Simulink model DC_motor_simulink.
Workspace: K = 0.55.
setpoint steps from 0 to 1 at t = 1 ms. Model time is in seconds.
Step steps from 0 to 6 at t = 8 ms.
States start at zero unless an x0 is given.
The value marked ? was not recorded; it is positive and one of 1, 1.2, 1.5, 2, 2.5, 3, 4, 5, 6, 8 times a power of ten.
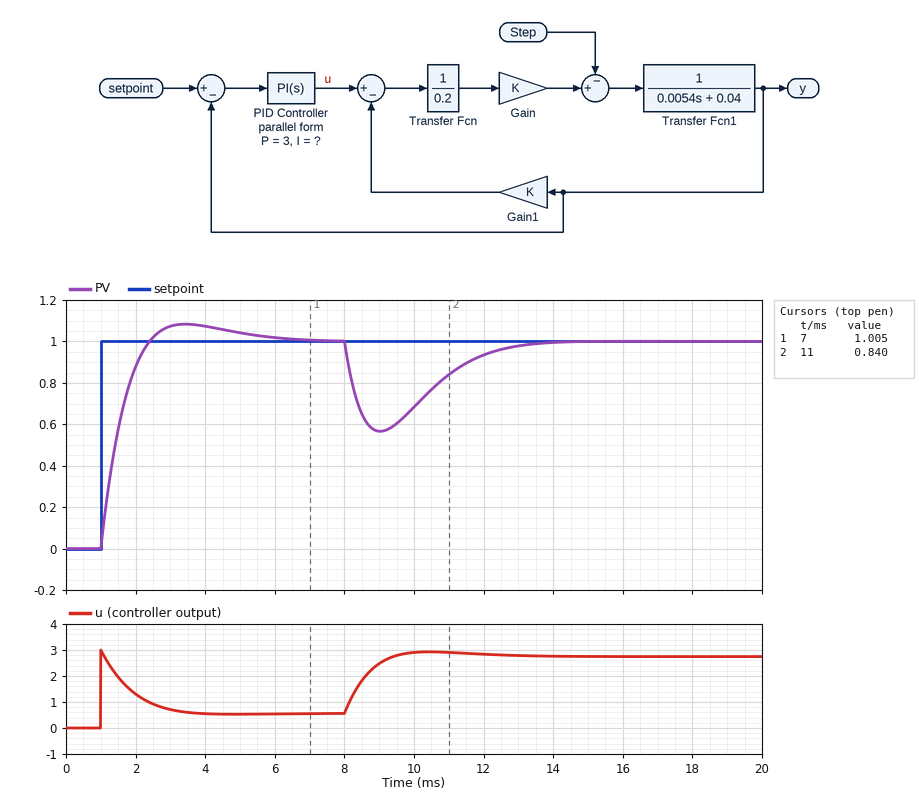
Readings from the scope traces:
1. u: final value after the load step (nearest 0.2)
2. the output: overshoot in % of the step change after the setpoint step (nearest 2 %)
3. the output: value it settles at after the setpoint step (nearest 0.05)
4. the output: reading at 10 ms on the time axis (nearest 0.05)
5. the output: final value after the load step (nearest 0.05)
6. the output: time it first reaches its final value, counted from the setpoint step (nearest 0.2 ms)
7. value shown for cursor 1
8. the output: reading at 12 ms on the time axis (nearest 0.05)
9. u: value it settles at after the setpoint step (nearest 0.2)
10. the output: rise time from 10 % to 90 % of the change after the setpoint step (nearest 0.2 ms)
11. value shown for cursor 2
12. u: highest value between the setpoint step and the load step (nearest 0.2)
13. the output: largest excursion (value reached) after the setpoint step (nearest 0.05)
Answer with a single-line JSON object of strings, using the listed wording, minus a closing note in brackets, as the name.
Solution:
{"u: final value after the load step": "2.8", "the output: overshoot in % of the step change after the setpoint step": "8 %", "the output: value it settles at after the setpoint step": "1.00", "the output: reading at 10 ms on the time axis": "0.70", "the output: final value after the load step": "1.00", "the output: time it first reaches its final value, counted from the setpoint step": "1.4 ms", "value shown for cursor 1": "1.005", "the output: reading at 12 ms on the time axis": "0.95", "u: value it settles at after the setpoint step": "0.6", "the output: rise time from 10 % to 90 % of the change after the setpoint step": "1.0 ms", "value shown for cursor 2": "0.840", "u: highest value between the setpoint step and the load step": "3.0", "the output: largest excursion (value reached) after the setpoint step": "1.10"}
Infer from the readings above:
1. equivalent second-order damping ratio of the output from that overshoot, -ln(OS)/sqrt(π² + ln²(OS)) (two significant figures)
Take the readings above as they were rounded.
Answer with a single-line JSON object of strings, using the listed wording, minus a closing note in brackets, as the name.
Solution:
{"equivalent second-order damping ratio of the output from that overshoot, -ln(OS)/sqrt(π² + ln²(OS))": "0.63"}
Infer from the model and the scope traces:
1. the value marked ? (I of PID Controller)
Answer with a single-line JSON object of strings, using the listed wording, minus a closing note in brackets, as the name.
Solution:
{"the value marked ?": "2000"}
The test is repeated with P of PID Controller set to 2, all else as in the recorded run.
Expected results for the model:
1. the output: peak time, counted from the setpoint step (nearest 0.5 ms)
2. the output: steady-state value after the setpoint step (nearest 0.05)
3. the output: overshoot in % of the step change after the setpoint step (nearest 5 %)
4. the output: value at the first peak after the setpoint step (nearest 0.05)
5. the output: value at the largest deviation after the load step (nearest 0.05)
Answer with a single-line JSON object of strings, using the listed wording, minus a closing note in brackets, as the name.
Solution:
{"the output: peak time, counted from the setpoint step": "2.5 ms", "the output: steady-state value after the setpoint step": "1.00", "the output: overshoot in % of the step change after the setpoint step": "15 %", "the output: value at the first peak after the setpoint step": "1.15", "the output: value at the largest deviation after the load step": "0.45"}
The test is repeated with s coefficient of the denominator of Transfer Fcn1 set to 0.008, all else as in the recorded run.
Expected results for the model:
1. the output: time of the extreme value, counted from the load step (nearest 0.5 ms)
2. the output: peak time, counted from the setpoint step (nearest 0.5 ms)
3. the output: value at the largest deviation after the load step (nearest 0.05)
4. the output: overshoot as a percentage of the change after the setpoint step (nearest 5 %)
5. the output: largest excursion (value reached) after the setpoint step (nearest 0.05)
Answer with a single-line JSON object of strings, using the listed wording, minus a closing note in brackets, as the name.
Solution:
{"the output: time of the extreme value, counted from the load step": "1.5 ms", "the output: peak time, counted from the setpoint step": "3.0 ms", "the output: value at the largest deviation after the load step": "0.60", "the output: overshoot as a percentage of the change after the setpoint step": "15 %", "the output: largest excursion (value reached) after the setpoint step": "1.15"}
